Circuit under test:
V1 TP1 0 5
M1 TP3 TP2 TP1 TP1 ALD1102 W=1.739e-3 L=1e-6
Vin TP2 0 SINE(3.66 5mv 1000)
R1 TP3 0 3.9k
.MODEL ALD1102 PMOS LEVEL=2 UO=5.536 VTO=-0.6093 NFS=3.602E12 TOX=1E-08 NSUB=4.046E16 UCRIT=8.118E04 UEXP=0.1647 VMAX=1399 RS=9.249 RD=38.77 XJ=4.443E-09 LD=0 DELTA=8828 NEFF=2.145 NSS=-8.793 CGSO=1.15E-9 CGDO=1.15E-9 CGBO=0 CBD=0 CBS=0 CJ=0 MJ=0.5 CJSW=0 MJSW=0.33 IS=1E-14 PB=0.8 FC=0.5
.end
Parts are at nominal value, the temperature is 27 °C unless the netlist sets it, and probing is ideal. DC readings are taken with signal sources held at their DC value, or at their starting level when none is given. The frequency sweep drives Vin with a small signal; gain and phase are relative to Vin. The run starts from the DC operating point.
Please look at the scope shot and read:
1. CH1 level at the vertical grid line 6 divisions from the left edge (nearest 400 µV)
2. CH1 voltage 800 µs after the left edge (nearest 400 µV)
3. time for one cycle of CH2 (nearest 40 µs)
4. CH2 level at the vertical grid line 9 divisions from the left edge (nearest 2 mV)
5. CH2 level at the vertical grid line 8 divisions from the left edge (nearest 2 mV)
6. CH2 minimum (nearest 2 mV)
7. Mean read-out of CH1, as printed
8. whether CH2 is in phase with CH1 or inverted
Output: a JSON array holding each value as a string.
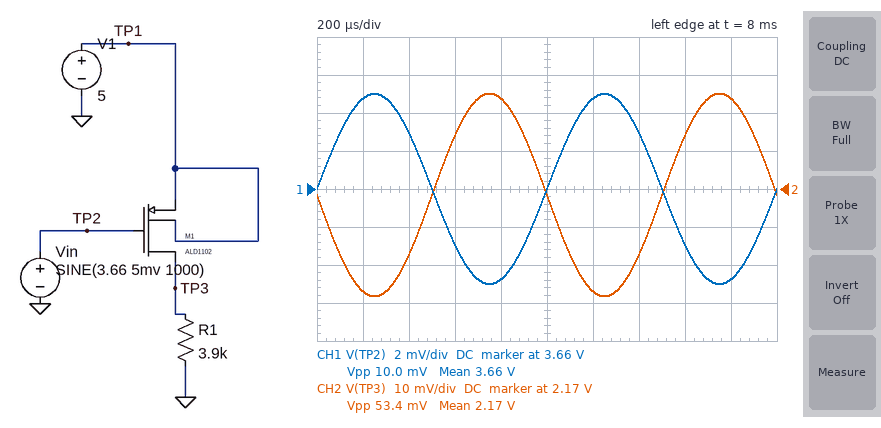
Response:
["3.6648 V", "3.6552 V", "1.00 ms", "2.194 V", "2.184 V", "2.142 V", "3.66 V", "inverted"]
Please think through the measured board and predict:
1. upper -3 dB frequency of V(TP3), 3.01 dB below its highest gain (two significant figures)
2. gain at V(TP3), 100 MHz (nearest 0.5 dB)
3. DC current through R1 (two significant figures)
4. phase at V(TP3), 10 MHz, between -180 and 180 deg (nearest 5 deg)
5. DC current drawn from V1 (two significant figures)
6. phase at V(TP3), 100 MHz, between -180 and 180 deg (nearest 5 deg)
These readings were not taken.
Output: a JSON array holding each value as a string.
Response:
["23 MHz", "4.0 dB", "560 µA", "150 deg", "560 µA", "60 deg"]
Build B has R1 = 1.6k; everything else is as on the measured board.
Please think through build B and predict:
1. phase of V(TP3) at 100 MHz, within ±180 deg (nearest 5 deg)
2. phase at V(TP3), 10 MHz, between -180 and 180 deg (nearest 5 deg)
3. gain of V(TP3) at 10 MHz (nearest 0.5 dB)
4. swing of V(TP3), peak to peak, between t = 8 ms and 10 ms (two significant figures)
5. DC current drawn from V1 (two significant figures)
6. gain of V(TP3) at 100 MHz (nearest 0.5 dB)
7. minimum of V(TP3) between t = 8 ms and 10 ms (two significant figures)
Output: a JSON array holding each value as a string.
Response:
["75 deg", "165 deg", "7.5 dB", "25 mV", "590 µA", "3.0 dB", "930 mV"]
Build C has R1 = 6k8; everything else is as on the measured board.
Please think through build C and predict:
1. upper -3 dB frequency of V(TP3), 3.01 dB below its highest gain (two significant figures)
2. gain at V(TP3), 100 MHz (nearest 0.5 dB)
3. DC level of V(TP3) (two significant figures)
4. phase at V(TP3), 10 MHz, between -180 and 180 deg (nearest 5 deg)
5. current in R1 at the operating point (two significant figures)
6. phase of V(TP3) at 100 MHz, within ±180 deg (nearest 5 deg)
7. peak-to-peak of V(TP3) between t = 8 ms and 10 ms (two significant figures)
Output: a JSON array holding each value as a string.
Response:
["15 MHz", "3.5 dB", "3.5 V", "140 deg", "520 µA", "55 deg", "77 mV"]
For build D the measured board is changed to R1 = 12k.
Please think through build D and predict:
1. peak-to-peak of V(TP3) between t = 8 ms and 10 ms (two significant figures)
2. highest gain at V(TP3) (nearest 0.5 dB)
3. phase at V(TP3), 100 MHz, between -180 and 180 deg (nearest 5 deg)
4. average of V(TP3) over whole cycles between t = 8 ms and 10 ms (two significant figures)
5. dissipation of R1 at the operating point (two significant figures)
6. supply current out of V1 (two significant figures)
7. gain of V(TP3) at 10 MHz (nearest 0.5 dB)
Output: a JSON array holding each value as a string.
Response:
["9.0 mV", "0 dB", "35 deg", "4.7 V", "1.8 mW", "390 µA", "-3.0 dB"]
